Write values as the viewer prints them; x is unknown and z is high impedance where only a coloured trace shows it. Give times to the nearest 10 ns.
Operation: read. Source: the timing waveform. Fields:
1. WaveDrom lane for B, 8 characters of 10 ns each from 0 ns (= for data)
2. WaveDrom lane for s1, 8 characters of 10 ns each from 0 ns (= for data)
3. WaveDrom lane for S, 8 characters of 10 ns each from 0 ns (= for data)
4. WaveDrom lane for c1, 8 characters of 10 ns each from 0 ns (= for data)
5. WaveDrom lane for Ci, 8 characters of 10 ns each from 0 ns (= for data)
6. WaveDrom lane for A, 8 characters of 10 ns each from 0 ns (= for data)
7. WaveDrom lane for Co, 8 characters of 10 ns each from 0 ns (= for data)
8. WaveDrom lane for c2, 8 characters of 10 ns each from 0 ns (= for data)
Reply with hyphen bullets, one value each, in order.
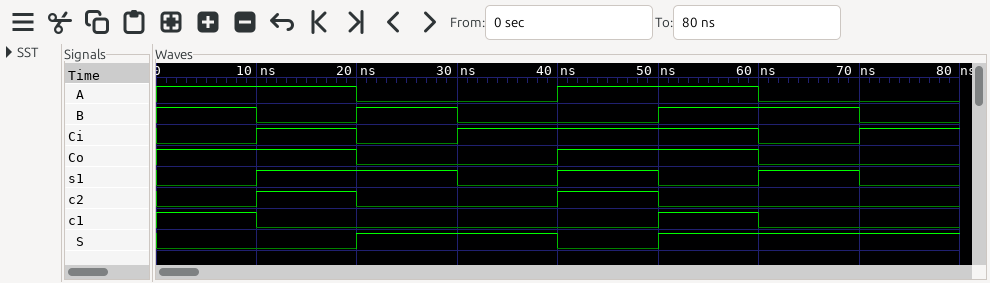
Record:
- {name: 'B', wave: '1010.1.0'}
- {name: 's1', wave: '01.01010'}
- {name: 'S', wave: '0.1.01..'}
- {name: 'c1', wave: '10...10.'}
- {name: 'Ci', wave: '0101..01'}
- {name: 'A', wave: '1.0.1.0.'}
- {name: 'Co', wave: '1.0.1.0.'}
- {name: 'c2', wave: '010.10..'}
